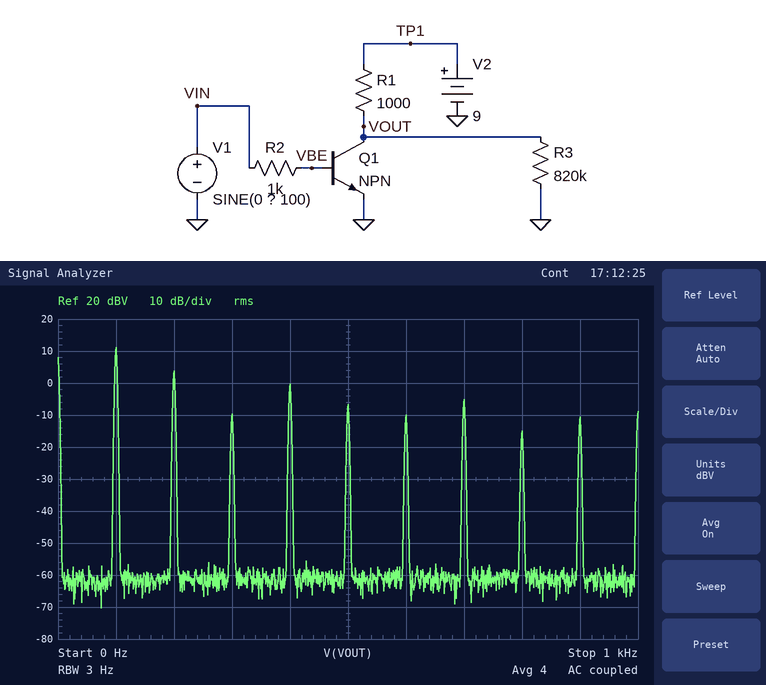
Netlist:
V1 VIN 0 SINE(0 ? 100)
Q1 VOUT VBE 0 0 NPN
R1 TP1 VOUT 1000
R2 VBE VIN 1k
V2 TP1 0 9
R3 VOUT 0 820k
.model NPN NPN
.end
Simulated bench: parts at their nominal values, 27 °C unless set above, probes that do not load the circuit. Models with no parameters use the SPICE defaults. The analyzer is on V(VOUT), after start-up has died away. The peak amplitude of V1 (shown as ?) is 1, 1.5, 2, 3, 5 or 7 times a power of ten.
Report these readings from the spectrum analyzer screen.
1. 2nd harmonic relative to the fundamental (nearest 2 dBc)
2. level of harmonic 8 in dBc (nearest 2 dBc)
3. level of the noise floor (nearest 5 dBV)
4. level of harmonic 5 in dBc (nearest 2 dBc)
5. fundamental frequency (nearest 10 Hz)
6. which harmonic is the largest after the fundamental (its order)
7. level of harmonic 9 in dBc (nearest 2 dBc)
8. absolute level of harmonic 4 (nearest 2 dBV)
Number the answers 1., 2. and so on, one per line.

1. -8 dBc
2. -26 dBc
3. -60 dBV
4. -18 dBc
5. 100 Hz
6. 2
7. -22 dBc
8. 0 dBV
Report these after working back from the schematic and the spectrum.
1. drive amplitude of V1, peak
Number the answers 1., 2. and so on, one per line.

1. 2 V
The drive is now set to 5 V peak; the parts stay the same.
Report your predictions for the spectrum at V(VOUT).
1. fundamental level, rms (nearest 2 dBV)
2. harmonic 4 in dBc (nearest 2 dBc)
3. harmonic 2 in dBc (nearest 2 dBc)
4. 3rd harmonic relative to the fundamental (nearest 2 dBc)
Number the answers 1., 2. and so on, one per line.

1. 12 dBV
2. -16 dBc
3. -16 dBc
4. -10 dBc
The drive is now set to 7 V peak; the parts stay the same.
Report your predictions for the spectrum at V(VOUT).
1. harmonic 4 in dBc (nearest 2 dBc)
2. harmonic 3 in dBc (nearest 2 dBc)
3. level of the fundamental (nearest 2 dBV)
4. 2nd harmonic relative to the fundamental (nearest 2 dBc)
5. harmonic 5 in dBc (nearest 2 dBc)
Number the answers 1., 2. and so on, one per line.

1. -18 dBc
2. -10 dBc
3. 12 dBV
4. -18 dBc
5. -16 dBc
